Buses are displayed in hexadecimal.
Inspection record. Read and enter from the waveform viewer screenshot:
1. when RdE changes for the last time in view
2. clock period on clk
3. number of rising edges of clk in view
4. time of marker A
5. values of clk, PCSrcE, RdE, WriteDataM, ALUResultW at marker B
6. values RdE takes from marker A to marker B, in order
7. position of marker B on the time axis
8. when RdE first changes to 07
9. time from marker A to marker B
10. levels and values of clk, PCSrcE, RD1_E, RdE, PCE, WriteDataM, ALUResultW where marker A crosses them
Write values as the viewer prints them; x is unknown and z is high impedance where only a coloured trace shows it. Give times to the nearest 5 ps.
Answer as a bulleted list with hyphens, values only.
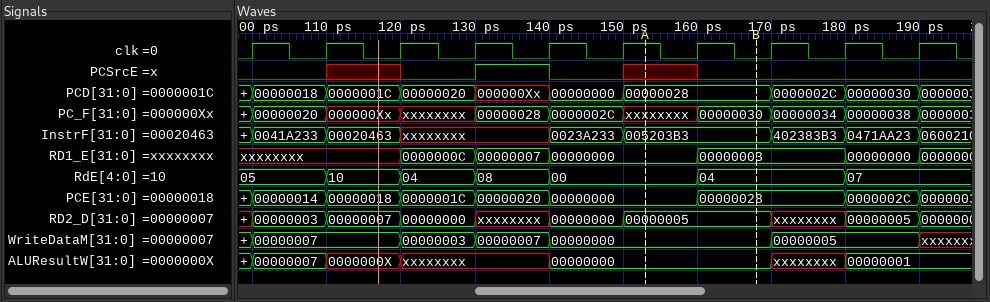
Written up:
- 180 ps
- 10 ps
- 10
- 155 ps
- clk=0, PCSrcE=0, RdE=04, WriteDataM=00000000, ALUResultW=00000000
- 00, 04
- 170 ps
- 180 ps
- 15 ps
- clk=1, PCSrcE=x, RD1_E=00000000, RdE=00, PCE=00000000, WriteDataM=00000000, ALUResultW=00000000
